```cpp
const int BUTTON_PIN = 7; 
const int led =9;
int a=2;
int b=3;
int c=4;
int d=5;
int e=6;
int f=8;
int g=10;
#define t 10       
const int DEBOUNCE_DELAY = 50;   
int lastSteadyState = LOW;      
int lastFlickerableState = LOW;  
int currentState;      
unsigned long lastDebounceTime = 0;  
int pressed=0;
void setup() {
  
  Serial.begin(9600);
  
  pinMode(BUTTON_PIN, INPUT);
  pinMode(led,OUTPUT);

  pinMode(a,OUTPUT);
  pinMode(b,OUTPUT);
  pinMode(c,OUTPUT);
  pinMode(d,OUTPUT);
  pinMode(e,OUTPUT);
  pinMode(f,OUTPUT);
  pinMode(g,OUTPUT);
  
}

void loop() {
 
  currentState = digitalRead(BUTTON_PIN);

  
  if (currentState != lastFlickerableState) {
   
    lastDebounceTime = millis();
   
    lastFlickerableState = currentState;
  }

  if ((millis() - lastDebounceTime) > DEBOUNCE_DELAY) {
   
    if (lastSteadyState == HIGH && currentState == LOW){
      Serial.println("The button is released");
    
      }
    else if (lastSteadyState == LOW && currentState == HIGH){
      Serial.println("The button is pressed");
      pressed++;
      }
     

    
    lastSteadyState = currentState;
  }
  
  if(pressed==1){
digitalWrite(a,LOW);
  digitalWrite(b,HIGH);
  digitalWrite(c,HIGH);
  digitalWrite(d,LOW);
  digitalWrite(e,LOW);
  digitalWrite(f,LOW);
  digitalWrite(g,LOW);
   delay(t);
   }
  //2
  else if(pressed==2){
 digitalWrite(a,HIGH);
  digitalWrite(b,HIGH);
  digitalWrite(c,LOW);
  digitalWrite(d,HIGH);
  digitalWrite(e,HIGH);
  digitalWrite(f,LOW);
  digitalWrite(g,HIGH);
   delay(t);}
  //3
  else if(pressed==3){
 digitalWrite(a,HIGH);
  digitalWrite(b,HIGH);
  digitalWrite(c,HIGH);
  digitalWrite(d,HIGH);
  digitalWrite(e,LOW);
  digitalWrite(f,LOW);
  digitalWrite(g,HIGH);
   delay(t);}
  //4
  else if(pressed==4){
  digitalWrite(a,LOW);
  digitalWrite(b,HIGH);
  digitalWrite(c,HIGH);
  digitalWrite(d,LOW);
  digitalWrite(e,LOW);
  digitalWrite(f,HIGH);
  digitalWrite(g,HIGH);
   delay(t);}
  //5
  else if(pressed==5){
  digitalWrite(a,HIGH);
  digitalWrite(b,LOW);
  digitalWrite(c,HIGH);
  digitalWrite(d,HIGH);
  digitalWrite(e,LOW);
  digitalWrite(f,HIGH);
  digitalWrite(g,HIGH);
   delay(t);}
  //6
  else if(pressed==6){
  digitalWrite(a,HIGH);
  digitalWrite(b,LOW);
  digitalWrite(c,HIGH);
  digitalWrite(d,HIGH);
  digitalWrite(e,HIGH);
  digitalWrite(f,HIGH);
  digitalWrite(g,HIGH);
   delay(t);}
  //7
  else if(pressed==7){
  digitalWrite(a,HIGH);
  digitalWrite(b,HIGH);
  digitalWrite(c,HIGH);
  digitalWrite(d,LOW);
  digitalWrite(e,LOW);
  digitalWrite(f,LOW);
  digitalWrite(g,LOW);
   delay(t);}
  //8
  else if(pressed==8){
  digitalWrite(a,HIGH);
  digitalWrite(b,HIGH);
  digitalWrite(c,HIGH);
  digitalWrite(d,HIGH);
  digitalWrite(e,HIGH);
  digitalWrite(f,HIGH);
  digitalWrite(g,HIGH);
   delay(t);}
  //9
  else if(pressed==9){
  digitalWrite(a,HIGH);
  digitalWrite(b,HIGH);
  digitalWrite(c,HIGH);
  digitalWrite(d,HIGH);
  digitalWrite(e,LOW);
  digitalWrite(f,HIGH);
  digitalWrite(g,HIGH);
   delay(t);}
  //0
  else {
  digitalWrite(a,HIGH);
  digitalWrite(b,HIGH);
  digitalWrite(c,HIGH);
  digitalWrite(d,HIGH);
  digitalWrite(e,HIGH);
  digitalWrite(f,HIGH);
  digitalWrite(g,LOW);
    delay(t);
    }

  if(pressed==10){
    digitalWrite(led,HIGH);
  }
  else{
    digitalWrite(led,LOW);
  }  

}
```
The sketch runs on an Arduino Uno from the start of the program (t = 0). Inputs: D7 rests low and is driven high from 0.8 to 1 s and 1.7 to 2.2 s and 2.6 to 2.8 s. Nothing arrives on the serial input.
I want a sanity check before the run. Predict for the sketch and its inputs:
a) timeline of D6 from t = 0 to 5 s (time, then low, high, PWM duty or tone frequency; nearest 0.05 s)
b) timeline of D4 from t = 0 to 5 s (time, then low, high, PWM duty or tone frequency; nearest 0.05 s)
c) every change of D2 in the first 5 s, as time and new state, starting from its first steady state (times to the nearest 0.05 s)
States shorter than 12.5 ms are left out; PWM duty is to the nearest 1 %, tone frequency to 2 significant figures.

0 s high; 0.85 s low; 1.75 s high; 2.65 s low
0 s high; 1.75 s low; 2.65 s high
0 s high; 0.85 s low; 1.75 s high
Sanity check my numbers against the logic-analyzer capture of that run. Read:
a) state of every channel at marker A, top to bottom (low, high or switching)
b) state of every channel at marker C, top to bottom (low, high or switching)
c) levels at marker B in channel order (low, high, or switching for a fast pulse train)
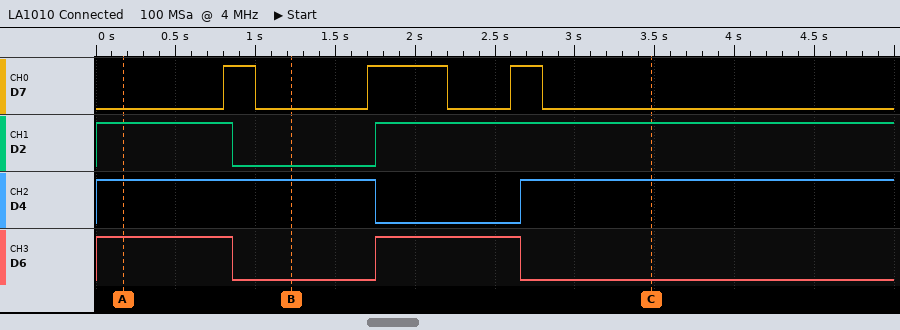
D7 low, D2 high, D4 high, D6 high
D7 low, D2 high, D4 high, D6 low
D7 low, D2 low, D4 high, D6 low
